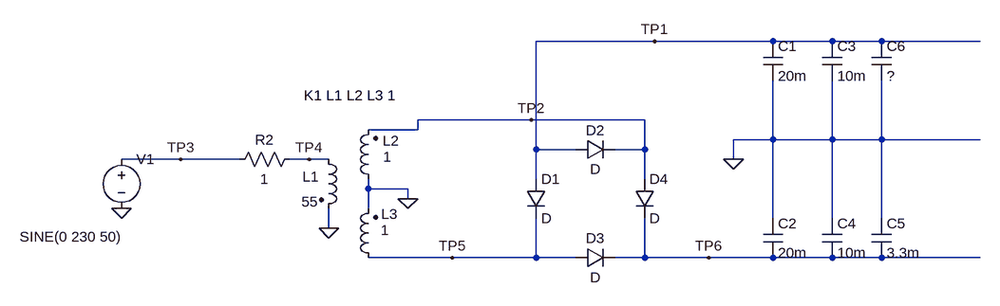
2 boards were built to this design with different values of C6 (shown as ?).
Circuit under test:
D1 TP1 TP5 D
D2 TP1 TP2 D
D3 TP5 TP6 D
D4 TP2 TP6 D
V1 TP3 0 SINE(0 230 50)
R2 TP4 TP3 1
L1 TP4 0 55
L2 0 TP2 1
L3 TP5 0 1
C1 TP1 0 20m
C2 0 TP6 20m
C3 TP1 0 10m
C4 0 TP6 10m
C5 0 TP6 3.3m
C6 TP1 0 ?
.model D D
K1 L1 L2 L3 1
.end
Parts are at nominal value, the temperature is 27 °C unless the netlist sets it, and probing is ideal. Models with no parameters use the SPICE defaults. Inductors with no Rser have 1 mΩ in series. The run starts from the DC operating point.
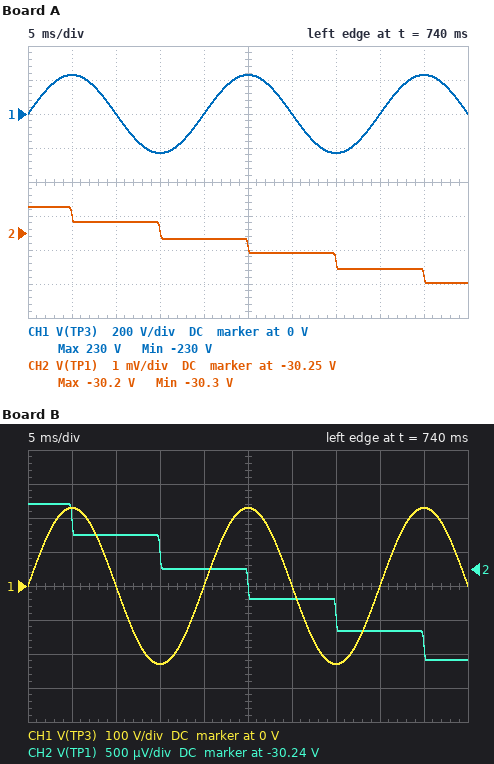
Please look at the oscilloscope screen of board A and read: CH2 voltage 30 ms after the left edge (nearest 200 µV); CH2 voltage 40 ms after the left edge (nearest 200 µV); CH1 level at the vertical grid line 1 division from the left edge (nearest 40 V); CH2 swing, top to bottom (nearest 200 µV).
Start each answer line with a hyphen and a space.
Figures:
- -30.2496 V
- -30.2500 V
- 240 V
- 2.2 mV
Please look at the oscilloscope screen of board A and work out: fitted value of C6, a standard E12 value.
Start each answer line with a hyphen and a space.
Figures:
- 2.2 mF
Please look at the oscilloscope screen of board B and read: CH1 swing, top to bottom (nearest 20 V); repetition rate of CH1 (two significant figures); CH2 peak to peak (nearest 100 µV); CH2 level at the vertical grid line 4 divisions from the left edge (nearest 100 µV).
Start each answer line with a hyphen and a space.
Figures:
- 460 V
- 50 Hz
- 2.3 mV
- -30.2425 V
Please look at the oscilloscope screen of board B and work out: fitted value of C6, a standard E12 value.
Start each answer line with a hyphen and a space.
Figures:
- 10 mF
